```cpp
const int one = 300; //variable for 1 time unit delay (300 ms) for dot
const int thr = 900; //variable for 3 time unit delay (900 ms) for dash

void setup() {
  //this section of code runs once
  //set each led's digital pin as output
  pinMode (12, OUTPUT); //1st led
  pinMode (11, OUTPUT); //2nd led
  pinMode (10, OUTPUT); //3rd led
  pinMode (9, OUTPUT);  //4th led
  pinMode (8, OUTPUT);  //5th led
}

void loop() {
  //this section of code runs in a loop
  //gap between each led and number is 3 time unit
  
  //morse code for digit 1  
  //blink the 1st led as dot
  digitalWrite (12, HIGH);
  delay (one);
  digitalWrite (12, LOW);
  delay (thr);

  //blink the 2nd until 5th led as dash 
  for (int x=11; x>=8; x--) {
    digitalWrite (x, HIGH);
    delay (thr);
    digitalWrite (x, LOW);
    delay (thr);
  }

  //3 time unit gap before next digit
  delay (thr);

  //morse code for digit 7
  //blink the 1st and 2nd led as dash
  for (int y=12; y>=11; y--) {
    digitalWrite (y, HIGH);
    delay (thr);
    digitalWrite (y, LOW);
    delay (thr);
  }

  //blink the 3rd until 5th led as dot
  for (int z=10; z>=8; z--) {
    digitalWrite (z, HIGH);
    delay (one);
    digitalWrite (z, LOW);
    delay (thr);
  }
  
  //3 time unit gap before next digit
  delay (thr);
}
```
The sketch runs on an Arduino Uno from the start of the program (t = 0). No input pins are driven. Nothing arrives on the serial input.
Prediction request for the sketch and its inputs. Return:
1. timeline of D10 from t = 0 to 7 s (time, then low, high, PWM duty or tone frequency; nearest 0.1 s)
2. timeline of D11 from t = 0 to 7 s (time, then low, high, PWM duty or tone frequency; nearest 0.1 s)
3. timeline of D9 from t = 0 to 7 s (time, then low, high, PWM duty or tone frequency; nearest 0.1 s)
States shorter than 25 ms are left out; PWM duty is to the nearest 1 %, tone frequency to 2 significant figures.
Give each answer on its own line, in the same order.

0 s low; 3 s high; 3.9 s low
0 s low; 1.2 s high; 2.1 s low
0 s low; 4.8 s high; 5.7 s low
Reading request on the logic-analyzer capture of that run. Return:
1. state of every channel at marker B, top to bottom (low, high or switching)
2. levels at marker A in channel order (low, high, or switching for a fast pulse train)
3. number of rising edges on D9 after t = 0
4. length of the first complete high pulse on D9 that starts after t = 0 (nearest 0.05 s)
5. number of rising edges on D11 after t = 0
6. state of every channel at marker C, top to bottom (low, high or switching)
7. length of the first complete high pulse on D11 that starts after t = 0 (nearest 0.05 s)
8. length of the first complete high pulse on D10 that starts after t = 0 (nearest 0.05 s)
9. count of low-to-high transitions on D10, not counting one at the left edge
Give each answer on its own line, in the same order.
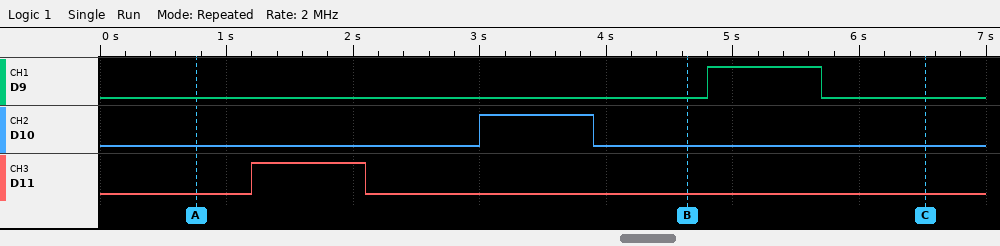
D9 low, D10 low, D11 low
D9 low, D10 low, D11 low
1
0.90 s
1
D9 low, D10 low, D11 low
0.90 s
0.90 s
1
